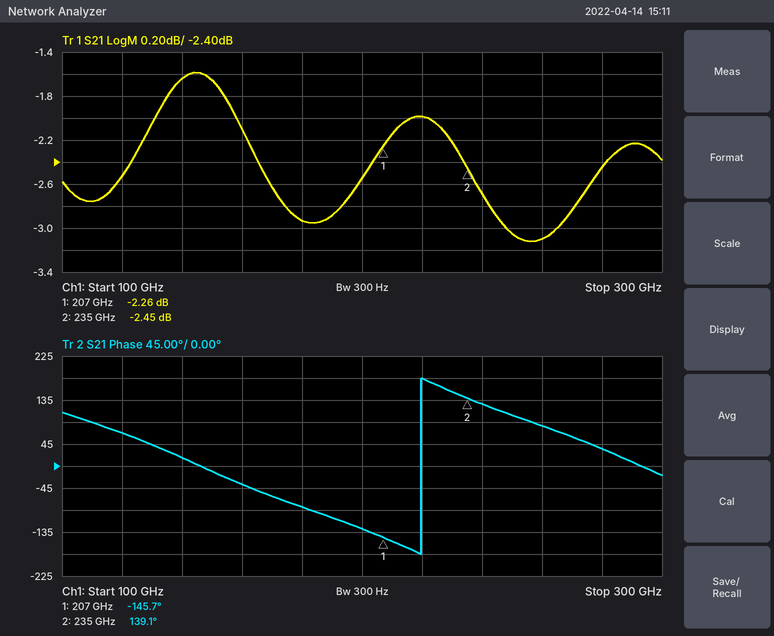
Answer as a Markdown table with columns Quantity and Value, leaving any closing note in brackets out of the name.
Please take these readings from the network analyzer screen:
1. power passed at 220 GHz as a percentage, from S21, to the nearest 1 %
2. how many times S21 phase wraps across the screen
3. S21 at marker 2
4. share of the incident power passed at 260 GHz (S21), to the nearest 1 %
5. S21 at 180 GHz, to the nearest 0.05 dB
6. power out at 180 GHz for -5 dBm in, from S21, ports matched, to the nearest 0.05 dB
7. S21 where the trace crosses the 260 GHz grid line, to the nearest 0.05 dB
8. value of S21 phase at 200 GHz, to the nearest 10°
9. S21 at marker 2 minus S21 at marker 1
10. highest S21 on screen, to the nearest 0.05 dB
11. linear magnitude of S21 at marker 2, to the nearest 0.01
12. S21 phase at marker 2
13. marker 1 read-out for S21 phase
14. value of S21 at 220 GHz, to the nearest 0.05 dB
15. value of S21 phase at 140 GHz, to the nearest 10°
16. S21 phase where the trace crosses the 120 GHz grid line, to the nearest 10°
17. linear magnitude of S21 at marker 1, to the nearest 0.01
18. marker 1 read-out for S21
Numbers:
| Quantity | Value |
|---|---|
| power passed at 220 GHz as a percentage, from S21, to the nearest 1 % | 63 % |
| how many times S21 phase wraps across the screen | 1 |
| S21 at marker 2 | -2.45 dB |
| share of the incident power passed at 260 GHz (S21), to the nearest 1 % | 49 % |
| S21 at 180 GHz, to the nearest 0.05 dB | -2.95 dB |
| power out at 180 GHz for -5 dBm in, from S21, ports matched, to the nearest 0.05 dB | -7.95 dBm |
| S21 where the trace crosses the 260 GHz grid line, to the nearest 0.05 dB | -3.10 dB |
| value of S21 phase at 200 GHz, to the nearest 10° | -130° |
| S21 at marker 2 minus S21 at marker 1 | -0.19 dB |
| highest S21 on screen, to the nearest 0.05 dB | -1.60 dB |
| linear magnitude of S21 at marker 2, to the nearest 0.01 | 0.75 |
| S21 phase at marker 2 | 139.1° |
| marker 1 read-out for S21 phase | -145.7° |
| value of S21 at 220 GHz, to the nearest 0.05 dB | -2.00 dB |
| value of S21 phase at 140 GHz, to the nearest 10° | 20° |
| S21 phase where the trace crosses the 120 GHz grid line, to the nearest 10° | 70° |
| linear magnitude of S21 at marker 1, to the nearest 0.01 | 0.77 |
| marker 1 read-out for S21 | -2.26 dB |
